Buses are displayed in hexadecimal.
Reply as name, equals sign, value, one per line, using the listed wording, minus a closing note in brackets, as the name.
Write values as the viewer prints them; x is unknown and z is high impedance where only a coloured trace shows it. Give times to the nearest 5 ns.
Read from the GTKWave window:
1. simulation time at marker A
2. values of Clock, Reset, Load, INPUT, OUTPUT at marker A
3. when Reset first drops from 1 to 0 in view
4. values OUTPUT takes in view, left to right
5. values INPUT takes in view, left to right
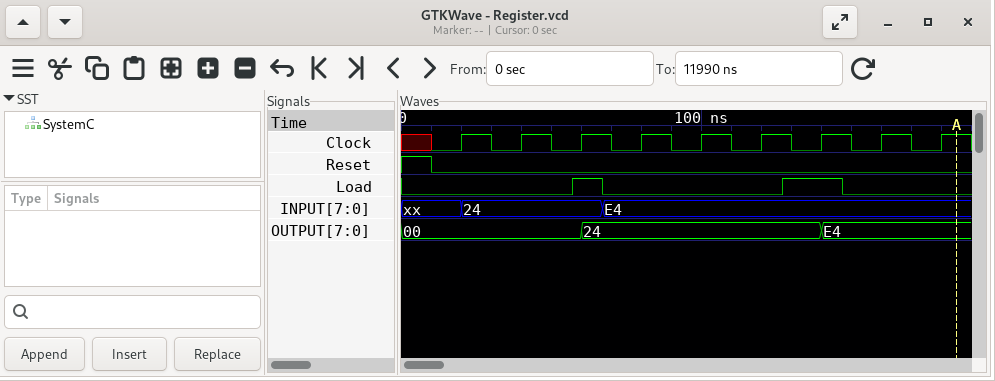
simulation time at marker A = 185 ns
values of Clock, Reset, Load, INPUT, OUTPUT at marker A = Clock=1, Reset=0, Load=0, INPUT=E4, OUTPUT=E4
when Reset first drops from 1 to 0 in view = 10 ns
values OUTPUT takes in view, left to right = 00, 24, E4
values INPUT takes in view, left to right = xx, 24, E4
